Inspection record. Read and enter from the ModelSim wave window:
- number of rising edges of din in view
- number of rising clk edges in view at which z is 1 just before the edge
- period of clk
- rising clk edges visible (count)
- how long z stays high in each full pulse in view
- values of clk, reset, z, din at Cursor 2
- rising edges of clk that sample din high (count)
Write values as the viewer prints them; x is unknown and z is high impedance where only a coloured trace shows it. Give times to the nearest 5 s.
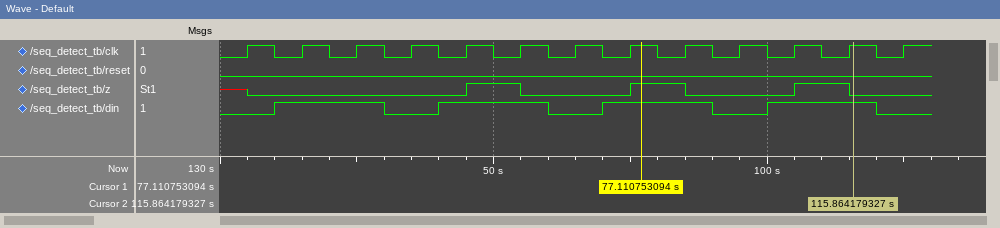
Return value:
4
3
10 s
13
10 s, 10 s, 10 s
clk=1, reset=0, z=0, din=1
8
